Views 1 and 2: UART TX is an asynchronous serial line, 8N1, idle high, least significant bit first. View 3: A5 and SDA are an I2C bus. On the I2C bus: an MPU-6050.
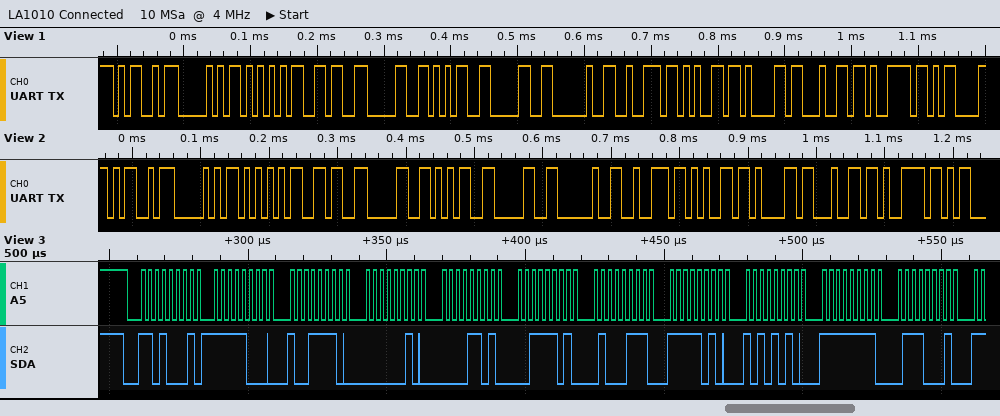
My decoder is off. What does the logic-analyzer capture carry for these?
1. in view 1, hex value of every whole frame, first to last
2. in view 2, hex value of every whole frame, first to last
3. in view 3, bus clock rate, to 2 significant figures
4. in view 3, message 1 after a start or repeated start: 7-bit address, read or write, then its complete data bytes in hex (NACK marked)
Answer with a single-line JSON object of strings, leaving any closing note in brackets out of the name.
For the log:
{"in view 1, hex value of every whole frame, first to last": "4D 50 55 36 30 35 30 20 72 65 61 64 79 0D", "in view 2, hex value of every whole frame, first to last": "4D 50 55 36 30 35 30 20 72 65 61 64 79", "in view 3, bus clock rate, to 2 significant figures": "400 kHz", "in view 3, message 1 after a start or repeated start: 7-bit address, read or write, then its complete data bytes in hex": "0x68 read: F8 9E 02 0D 3D 47 FA AA FF 71"}
